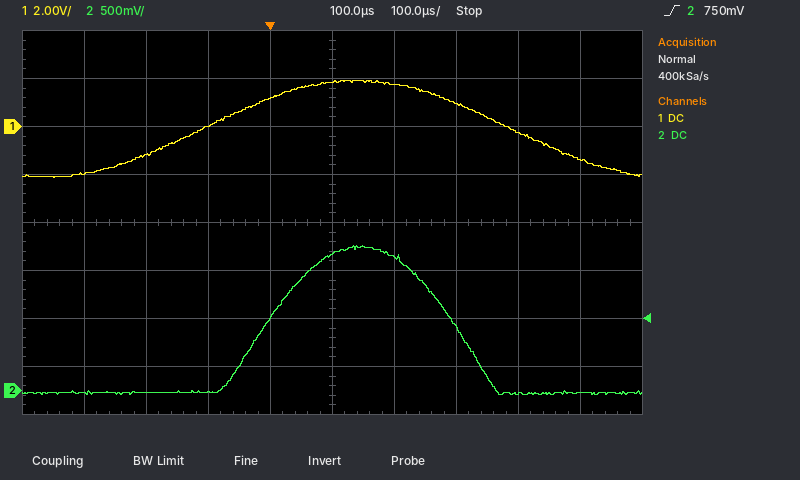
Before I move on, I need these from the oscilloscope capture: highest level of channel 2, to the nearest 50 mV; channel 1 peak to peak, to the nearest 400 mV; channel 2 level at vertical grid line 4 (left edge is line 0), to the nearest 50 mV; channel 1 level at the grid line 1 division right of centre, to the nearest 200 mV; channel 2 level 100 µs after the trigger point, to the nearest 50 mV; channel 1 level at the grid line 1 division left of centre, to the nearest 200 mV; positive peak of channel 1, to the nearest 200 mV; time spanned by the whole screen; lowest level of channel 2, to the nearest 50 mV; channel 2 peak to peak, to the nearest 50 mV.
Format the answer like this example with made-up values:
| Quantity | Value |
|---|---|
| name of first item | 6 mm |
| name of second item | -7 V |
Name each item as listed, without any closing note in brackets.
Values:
| Quantity | Value |
|---|---|
| highest level of channel 2, to the nearest 50 mV | 1.50 V |
| channel 1 peak to peak, to the nearest 400 mV | 4.0 V |
| channel 2 level at vertical grid line 4 (left edge is line 0), to the nearest 50 mV | 750 mV |
| channel 1 level at the grid line 1 division right of centre, to the nearest 200 mV | 1.8 V |
| channel 2 level 100 µs after the trigger point, to the nearest 50 mV | 1.40 V |
| channel 1 level at the grid line 1 division left of centre, to the nearest 200 mV | 1.2 V |
| positive peak of channel 1, to the nearest 200 mV | 2.0 V |
| time spanned by the whole screen | 1 ms |
| lowest level of channel 2, to the nearest 50 mV | -50 mV |
| channel 2 peak to peak, to the nearest 50 mV | 1.55 V |
